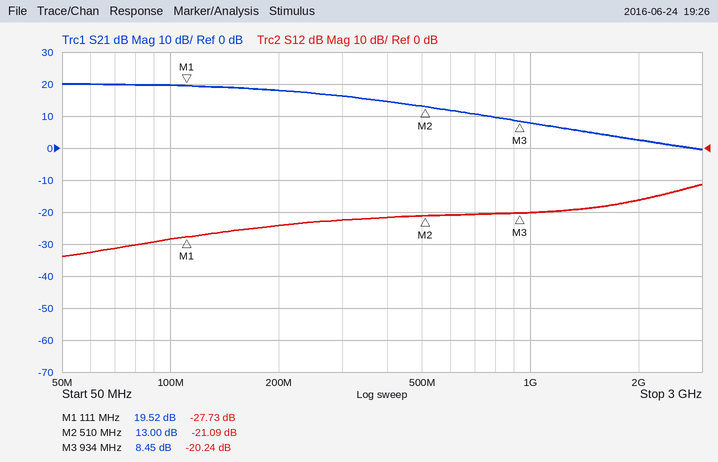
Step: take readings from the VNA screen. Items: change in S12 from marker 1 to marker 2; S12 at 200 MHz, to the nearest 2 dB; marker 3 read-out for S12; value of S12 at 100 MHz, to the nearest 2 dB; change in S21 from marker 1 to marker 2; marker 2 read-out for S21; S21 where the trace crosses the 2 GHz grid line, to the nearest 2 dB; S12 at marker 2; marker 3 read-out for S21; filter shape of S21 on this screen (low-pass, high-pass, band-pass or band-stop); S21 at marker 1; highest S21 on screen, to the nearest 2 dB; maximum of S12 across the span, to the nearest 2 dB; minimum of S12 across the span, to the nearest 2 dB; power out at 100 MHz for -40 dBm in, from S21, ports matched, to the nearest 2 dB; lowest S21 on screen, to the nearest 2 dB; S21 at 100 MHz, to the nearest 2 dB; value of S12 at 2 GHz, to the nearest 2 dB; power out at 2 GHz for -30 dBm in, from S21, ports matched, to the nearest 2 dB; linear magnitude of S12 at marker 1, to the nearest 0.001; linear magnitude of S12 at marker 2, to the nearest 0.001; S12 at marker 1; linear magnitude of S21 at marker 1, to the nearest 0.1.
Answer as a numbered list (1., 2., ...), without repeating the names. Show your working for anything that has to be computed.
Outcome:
1. -21.09 − (-27.73) = 6.64 dB
2. -24 dB
3. -20.24 dB
4. -28 dB
5. 13 − (19.52) = -6.52 dB
6. 13.00 dB
7. 2 dB
8. -21.09 dB
9. 8.45 dB
10. low-pass
11. 19.52 dB
12. 20 dB
13. -12 dB
14. -34 dB
15. -40 dBm + (20 dB) = -20 dBm
16. 0 dB
17. 20 dB
18. -16 dB
19. -30 dBm + (2 dB) = -28 dBm
20. 10^(-27.73/20) ≈ 0.041
21. 10^(-21.09/20) ≈ 0.088
22. -27.73 dB
23. 10^(19.52/20) ≈ 9.5
